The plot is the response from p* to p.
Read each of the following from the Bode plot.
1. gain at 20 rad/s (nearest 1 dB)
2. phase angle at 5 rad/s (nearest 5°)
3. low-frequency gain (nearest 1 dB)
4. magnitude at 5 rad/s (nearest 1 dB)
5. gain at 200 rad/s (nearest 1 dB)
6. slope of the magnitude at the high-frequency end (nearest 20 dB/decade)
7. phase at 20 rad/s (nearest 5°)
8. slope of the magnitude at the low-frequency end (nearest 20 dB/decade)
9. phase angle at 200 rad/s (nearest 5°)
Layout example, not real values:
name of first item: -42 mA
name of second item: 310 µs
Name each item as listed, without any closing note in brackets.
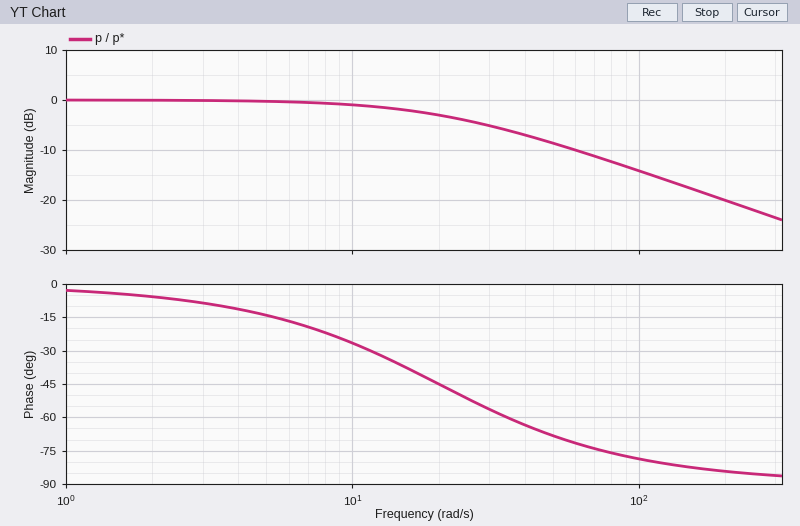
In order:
gain at 20 rad/s: -3 dB
phase angle at 5 rad/s: -15°
low-frequency gain: 0 dB
magnitude at 5 rad/s: 0 dB
gain at 200 rad/s: -20 dB
slope of the magnitude at the high-frequency end: -20 dB/decade
phase at 20 rad/s: -45°
slope of the magnitude at the low-frequency end: 0 dB/decade
phase angle at 200 rad/s: -85°
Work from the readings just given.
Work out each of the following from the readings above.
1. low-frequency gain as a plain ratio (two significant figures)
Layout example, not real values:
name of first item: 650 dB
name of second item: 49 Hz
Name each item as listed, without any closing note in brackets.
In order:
low-frequency gain as a plain ratio: 1.0
